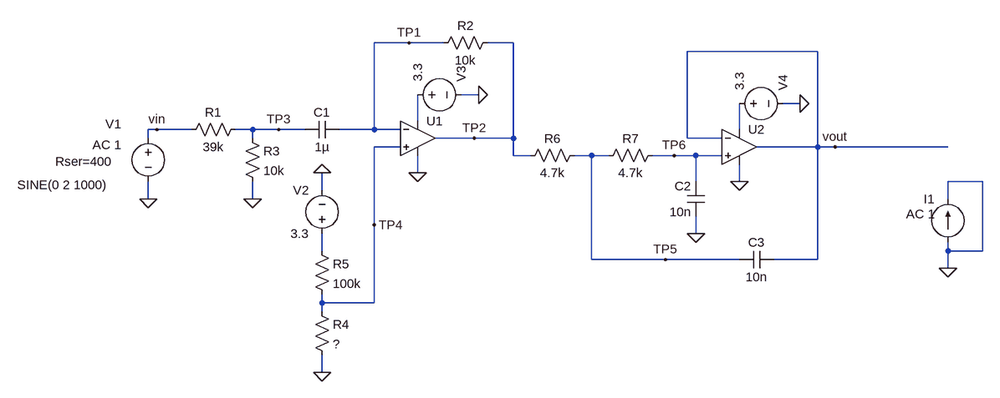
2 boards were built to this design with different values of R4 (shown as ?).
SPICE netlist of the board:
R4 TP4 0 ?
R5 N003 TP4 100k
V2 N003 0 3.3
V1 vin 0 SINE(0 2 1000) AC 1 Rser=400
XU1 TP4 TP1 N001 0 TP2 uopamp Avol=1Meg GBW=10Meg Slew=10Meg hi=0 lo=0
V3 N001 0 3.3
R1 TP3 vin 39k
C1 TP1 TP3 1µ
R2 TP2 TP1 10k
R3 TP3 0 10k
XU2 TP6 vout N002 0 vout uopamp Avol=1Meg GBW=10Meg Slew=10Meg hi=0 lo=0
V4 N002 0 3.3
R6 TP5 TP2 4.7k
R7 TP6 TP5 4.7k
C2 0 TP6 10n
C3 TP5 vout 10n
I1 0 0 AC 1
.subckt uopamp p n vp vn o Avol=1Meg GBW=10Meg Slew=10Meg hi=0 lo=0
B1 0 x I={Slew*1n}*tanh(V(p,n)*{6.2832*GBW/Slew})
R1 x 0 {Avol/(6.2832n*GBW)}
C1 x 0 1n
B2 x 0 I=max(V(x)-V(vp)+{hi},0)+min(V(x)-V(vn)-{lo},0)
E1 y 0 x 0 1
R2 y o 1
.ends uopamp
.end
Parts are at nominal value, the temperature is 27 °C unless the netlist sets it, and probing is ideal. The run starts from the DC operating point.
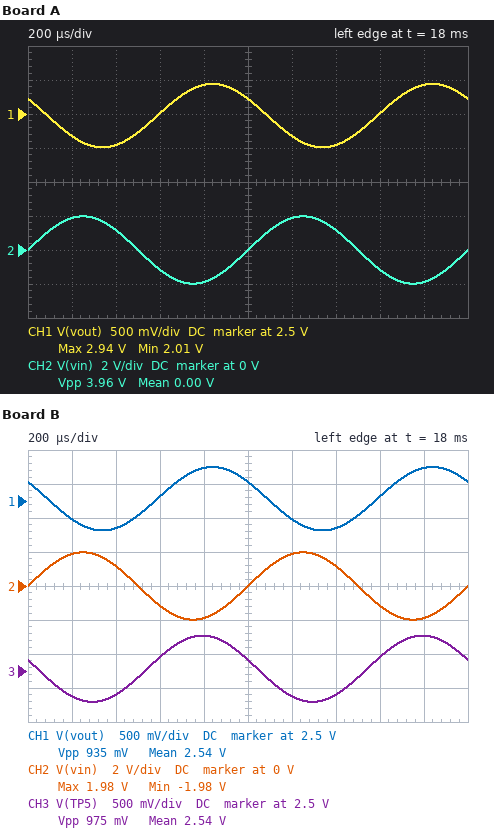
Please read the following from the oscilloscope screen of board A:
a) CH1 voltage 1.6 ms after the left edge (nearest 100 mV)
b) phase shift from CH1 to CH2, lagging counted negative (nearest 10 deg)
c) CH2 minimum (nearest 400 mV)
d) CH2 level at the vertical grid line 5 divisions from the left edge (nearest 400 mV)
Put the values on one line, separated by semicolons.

2.5 V; -150 deg; -2.0 V; 0 V
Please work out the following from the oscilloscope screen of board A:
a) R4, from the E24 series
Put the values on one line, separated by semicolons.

300 kΩ
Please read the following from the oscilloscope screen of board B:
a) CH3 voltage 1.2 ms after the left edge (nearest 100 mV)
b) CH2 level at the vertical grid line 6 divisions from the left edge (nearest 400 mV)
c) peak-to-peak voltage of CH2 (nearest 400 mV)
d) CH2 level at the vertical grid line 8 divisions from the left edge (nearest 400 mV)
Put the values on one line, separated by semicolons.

2.1 V; 2.0 V; 4.0 V; -1.2 V
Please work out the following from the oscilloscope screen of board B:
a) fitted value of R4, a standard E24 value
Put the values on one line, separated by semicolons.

330 kΩ
